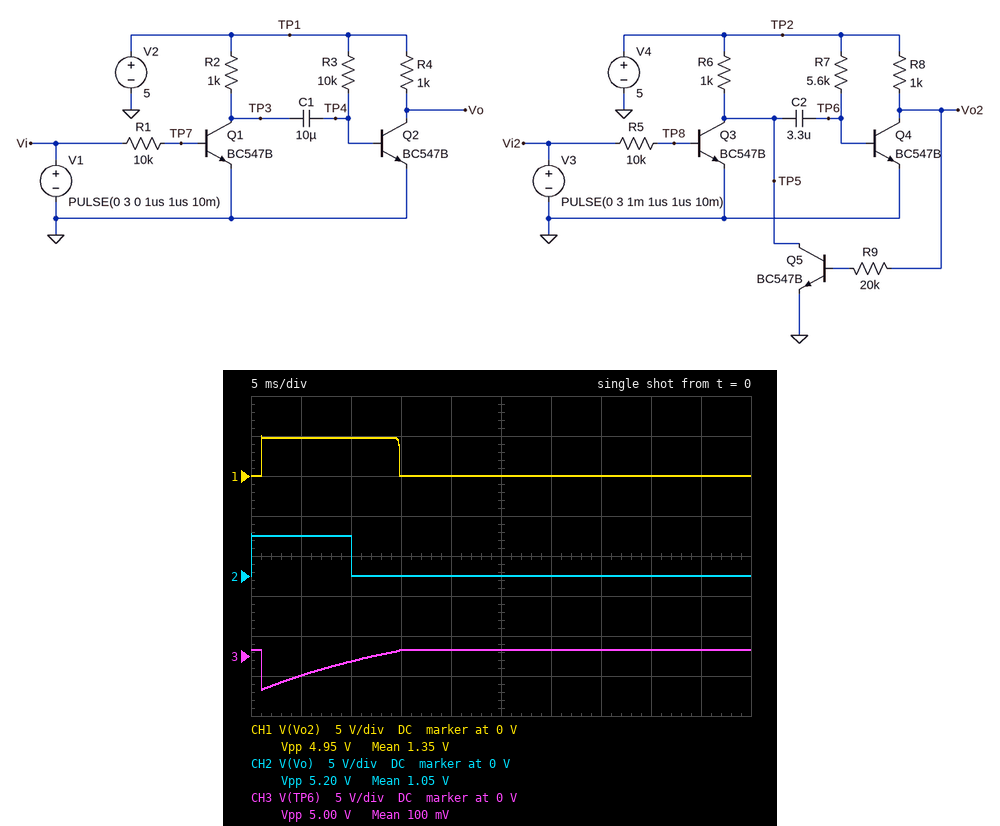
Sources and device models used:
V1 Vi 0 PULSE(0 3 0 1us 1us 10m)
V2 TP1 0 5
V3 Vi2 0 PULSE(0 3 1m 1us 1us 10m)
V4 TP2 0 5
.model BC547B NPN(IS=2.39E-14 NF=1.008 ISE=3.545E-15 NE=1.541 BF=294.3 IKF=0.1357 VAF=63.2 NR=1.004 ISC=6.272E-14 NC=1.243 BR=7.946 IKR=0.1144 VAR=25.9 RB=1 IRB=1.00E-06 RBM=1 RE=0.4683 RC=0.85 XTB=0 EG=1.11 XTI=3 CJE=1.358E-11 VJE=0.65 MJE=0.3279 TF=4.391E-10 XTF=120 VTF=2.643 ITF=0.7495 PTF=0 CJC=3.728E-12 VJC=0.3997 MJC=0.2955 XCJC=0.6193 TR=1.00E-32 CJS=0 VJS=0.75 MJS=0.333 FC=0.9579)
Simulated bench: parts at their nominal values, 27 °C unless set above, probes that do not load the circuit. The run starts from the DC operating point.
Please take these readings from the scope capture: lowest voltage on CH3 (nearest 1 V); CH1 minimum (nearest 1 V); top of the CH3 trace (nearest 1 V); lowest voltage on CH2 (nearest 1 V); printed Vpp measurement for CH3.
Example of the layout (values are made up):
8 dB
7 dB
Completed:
-4 V
0 V
1 V
0 V
5.00 V
